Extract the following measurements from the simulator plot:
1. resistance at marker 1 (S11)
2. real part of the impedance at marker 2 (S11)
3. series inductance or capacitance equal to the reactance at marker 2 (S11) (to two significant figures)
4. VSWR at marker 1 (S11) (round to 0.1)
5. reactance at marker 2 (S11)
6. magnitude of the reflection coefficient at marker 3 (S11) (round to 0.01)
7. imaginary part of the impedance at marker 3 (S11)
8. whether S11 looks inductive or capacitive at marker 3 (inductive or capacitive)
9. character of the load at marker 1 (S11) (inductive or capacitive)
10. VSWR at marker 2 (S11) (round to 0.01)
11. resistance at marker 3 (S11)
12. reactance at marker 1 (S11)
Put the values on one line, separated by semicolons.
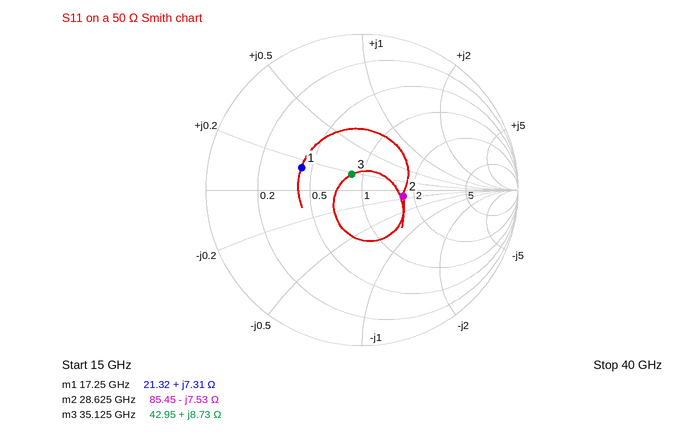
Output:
21.32 Ω; 85.45 Ω; 740 fF; 2.4; -7.53 Ω; 0.12; +8.73 Ω; inductive; inductive; 1.73; 42.95 Ω; +7.31 Ω
